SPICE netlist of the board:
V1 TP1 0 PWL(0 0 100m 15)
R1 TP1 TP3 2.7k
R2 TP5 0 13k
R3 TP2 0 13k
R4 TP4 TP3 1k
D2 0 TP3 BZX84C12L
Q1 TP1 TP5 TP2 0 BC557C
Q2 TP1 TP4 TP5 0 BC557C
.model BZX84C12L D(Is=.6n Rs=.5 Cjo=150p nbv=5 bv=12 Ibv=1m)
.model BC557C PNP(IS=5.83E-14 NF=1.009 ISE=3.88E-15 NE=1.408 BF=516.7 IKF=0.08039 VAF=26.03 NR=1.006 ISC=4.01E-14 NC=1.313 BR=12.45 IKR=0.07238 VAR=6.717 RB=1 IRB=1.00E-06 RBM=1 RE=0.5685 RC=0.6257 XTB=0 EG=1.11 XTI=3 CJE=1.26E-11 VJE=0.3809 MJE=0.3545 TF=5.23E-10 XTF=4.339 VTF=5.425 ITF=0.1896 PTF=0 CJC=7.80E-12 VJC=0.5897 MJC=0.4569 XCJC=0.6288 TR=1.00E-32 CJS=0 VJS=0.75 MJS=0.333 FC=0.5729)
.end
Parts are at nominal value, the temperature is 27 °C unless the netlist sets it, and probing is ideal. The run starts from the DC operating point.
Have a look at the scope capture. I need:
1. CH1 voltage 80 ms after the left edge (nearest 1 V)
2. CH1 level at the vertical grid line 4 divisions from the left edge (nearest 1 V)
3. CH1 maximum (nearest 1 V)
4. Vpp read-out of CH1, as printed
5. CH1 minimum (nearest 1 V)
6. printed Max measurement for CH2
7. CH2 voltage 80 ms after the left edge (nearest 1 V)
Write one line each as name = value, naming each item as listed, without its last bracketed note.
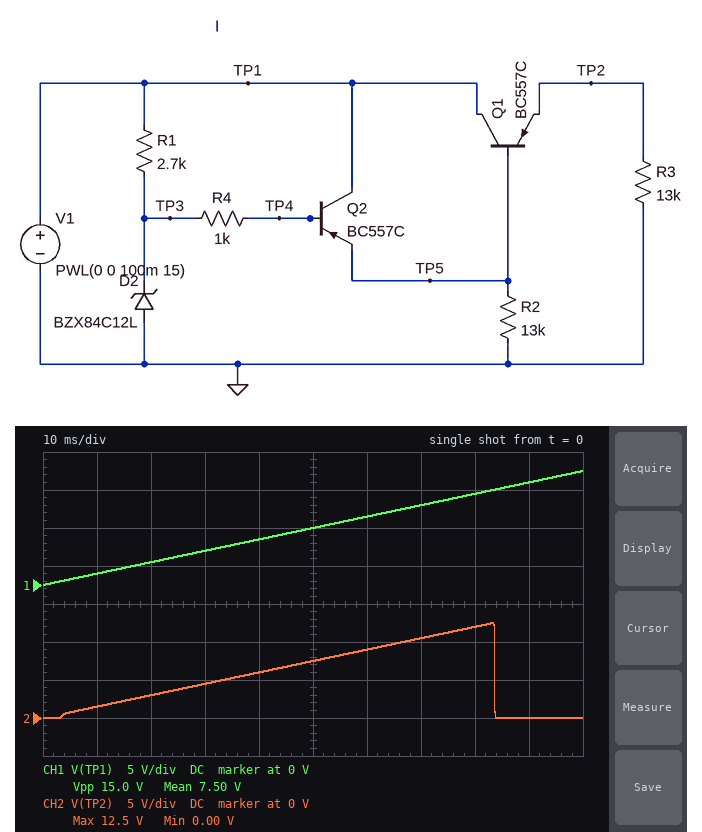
CH1 voltage 80 ms after the left edge = 12 V
CH1 level at the vertical grid line 4 divisions from the left edge = 6 V
CH1 maximum = 15 V
Vpp read-out of CH1, as printed = 15.0 V
CH1 minimum = 0 V
printed Max measurement for CH2 = 12.5 V
CH2 voltage 80 ms after the left edge = 12 V
